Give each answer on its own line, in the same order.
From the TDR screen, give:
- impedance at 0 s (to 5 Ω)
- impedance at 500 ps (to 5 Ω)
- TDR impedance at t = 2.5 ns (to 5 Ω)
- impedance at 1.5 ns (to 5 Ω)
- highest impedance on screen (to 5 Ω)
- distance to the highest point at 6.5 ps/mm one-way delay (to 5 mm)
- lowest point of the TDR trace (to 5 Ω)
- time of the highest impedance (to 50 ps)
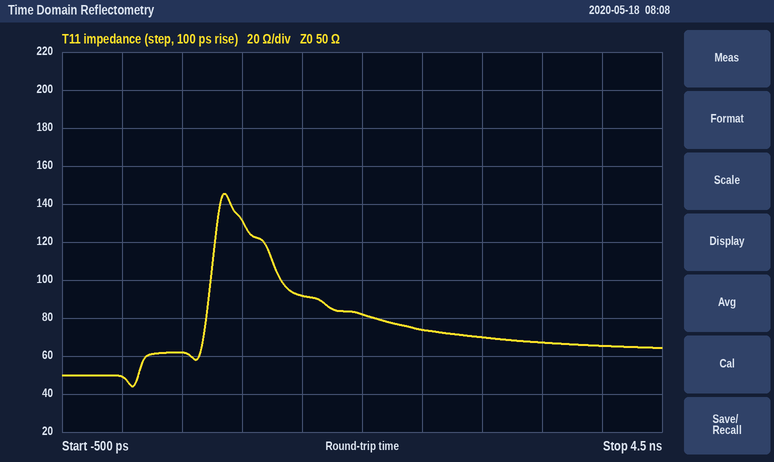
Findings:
50 Ω
60 Ω
75 Ω
90 Ω
145 Ω
65 mm
45 Ω
850 ps
